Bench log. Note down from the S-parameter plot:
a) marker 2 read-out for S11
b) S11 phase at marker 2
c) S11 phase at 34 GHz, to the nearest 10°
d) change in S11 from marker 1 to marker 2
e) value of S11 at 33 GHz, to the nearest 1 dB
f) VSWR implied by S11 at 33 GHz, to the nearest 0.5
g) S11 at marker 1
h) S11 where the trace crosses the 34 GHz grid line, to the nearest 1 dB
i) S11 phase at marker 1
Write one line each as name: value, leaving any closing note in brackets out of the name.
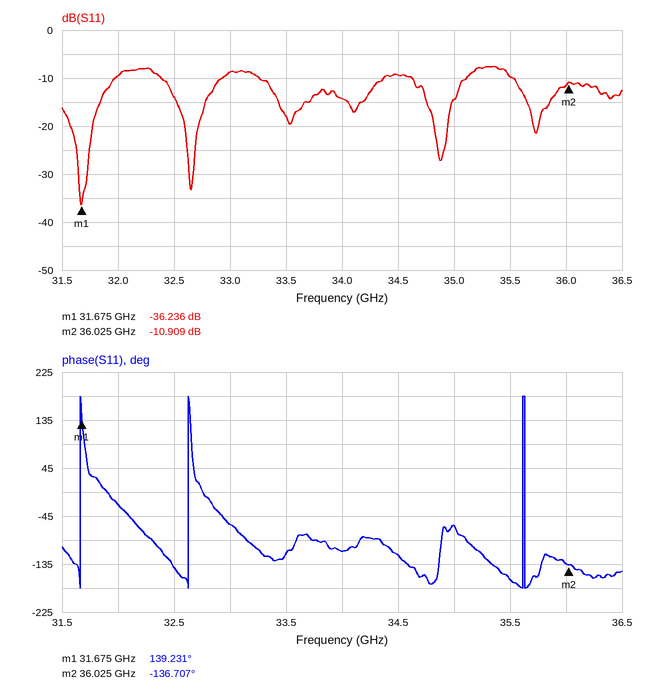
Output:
marker 2 read-out for S11: -10.909 dB
S11 phase at marker 2: -136.707°
S11 phase at 34 GHz, to the nearest 10°: -110°
change in S11 from marker 1 to marker 2: 25.327 dB
value of S11 at 33 GHz, to the nearest 1 dB: -9 dB
VSWR implied by S11 at 33 GHz, to the nearest 0.5: 2.0
S11 at marker 1: -36.236 dB
S11 where the trace crosses the 34 GHz grid line, to the nearest 1 dB: -14 dB
S11 phase at marker 1: 139.231°
